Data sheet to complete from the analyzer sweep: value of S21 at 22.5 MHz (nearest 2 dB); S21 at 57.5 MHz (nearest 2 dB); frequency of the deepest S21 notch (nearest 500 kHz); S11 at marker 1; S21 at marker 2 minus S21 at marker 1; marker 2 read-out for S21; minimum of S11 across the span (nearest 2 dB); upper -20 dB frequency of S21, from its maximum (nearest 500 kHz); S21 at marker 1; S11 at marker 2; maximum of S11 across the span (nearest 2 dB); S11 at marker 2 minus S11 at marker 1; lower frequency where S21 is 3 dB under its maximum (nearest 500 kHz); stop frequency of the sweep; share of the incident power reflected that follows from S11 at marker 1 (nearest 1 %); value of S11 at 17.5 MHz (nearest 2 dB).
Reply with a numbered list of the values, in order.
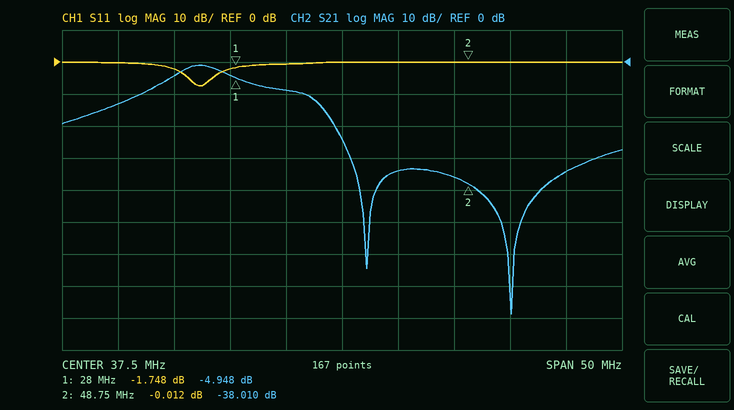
1. -4 dB
2. -34 dB
3. 52.5 MHz
4. -1.748 dB
5. -33.062 dB
6. -38.010 dB
7. -8 dB
8. 37.0 MHz
9. -4.948 dB
10. -0.012 dB
11. 0 dB
12. 1.736 dB
13. 22.5 MHz
14. 62.5 MHz
15. 67 %
16. 0 dB
